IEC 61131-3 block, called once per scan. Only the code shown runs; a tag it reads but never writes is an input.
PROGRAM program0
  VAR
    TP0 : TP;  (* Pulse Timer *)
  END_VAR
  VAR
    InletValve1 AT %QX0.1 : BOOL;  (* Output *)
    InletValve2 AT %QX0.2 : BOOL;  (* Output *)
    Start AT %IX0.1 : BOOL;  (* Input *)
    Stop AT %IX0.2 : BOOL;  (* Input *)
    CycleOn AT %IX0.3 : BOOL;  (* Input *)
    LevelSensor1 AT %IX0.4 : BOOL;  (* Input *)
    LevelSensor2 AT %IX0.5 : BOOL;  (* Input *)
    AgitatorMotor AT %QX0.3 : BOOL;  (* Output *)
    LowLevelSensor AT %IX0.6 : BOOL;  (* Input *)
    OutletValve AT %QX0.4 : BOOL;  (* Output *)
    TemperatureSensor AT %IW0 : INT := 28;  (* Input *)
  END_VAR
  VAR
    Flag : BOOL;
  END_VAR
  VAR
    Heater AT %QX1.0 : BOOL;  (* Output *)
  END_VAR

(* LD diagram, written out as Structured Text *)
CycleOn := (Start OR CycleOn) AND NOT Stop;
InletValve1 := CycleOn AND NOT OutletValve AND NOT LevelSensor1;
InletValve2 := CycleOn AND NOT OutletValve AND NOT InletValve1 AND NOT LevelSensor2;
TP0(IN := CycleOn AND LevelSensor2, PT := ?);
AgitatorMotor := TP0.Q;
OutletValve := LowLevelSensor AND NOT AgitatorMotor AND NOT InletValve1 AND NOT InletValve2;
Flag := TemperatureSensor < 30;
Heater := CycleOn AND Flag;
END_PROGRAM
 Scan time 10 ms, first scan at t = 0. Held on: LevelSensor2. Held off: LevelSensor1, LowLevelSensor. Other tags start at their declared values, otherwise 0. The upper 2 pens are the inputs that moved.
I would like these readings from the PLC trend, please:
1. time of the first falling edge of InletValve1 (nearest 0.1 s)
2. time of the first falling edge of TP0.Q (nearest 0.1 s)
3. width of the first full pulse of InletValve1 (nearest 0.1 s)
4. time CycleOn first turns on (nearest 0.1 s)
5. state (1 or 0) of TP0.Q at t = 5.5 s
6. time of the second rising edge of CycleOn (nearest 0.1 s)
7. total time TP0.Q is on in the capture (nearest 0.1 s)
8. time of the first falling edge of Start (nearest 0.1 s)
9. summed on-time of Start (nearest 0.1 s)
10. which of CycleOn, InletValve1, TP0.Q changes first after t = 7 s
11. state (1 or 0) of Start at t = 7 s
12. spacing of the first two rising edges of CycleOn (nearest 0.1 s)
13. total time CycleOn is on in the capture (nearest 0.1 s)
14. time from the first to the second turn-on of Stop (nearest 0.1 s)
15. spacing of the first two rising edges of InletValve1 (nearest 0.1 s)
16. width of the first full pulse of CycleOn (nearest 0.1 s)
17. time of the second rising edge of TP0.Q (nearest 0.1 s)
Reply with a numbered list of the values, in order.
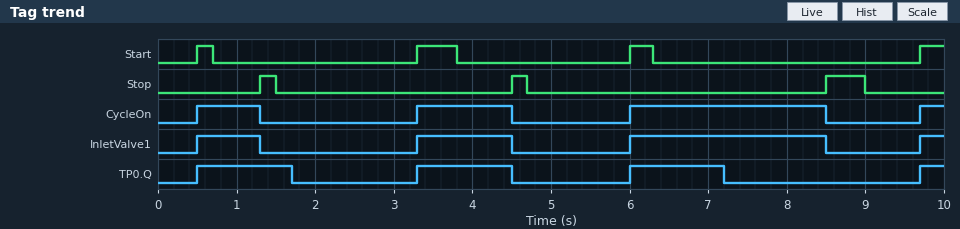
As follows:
1. 1.3 s
2. 1.7 s
3. 0.8 s
4. 0.5 s
5. 0
6. 3.3 s
7. 3.9 s
8. 0.7 s
9. 1.3 s
10. TP0.Q
11. 0
12. 2.8 s
13. 4.8 s
14. 3.2 s
15. 2.8 s
16. 0.8 s
17. 3.3 s
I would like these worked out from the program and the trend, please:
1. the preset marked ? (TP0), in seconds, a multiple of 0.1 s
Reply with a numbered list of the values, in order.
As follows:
1. 1.2 s
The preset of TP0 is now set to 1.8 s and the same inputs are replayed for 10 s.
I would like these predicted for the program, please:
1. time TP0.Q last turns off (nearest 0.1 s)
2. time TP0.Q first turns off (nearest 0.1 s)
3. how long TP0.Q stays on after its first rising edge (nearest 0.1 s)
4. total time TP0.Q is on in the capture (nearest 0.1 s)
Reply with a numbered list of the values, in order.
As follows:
1. 7.8 s
2. 2.3 s
3. 1.8 s
4. 5.7 s
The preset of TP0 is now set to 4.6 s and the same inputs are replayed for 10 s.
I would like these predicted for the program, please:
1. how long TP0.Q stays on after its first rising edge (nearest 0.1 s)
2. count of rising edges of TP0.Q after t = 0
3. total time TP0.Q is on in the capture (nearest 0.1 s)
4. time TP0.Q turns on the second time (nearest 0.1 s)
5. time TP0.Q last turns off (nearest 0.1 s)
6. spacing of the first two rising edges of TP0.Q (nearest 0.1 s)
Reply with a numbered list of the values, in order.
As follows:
1. 4.6 s
2. 2
3. 8.6 s
4. 6.0 s
5. 5.1 s
6. 5.5 s
